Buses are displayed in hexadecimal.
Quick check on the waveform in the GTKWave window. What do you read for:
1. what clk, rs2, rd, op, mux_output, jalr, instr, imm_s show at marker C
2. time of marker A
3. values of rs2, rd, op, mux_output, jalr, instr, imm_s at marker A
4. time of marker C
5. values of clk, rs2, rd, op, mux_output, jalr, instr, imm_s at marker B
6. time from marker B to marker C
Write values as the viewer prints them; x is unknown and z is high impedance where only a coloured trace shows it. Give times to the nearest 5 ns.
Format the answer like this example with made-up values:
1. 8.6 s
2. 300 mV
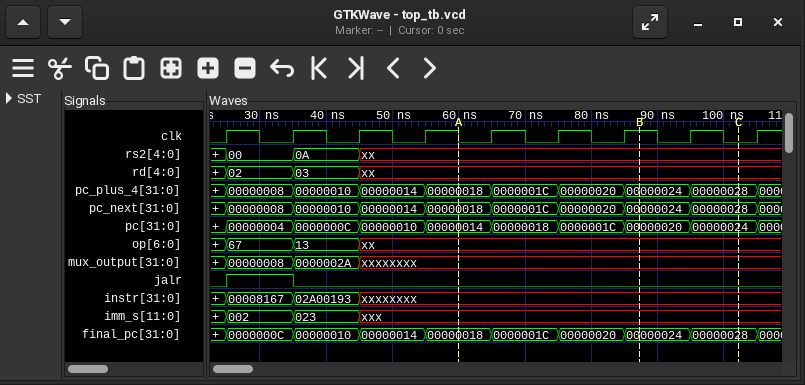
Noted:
1. clk=0, rs2=xx, rd=xx, op=xx, mux_output=xxxxxxxx, jalr=0, instr=xxxxxxxx, imm_s=xxx
2. 60 ns
3. rs2=xx, rd=xx, op=xx, mux_output=xxxxxxxx, jalr=0, instr=xxxxxxxx, imm_s=xxx
4. 100 ns
5. clk=1, rs2=xx, rd=xx, op=xx, mux_output=xxxxxxxx, jalr=0, instr=xxxxxxxx, imm_s=xxx
6. 15 ns
